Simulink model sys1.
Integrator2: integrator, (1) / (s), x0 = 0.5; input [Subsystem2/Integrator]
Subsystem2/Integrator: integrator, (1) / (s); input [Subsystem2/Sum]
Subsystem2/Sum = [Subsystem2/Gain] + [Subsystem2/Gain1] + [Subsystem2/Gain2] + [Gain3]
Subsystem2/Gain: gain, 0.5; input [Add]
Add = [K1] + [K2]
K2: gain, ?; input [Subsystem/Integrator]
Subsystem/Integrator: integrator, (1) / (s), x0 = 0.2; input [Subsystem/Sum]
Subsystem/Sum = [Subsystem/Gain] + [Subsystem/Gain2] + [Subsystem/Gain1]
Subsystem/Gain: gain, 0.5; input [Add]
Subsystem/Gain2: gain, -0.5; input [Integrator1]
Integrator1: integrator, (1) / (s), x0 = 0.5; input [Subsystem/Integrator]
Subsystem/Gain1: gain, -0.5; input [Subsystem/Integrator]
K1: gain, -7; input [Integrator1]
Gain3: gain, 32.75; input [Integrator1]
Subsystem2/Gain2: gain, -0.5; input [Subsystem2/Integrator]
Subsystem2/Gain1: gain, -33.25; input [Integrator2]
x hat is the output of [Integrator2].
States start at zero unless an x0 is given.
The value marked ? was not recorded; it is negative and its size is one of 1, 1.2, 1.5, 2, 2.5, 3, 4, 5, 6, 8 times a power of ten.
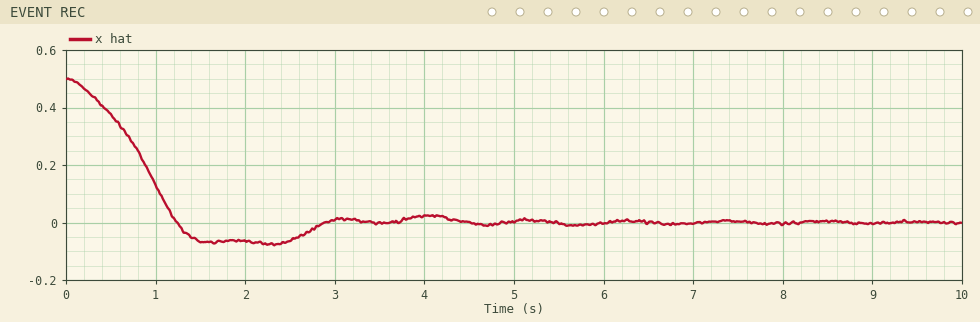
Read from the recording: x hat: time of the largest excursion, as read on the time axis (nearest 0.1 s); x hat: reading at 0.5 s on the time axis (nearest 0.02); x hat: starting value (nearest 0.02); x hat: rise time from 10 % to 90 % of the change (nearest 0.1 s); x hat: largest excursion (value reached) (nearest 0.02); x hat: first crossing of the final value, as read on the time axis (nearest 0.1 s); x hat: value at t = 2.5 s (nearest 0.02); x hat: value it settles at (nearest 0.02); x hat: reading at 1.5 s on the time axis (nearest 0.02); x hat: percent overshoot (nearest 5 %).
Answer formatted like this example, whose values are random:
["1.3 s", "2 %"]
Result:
["2.3 s", "0.38", "0.50", "0.9 s", "-0.08", "1.2 s", "-0.06", "0.00", "-0.06", "15 %"]
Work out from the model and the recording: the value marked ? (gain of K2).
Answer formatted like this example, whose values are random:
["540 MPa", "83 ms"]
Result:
["-3"]
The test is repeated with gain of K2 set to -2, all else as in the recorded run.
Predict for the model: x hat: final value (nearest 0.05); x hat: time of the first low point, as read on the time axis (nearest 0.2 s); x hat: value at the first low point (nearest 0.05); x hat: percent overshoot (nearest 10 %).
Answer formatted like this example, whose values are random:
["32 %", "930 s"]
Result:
["0.00", "1.6 s", "-0.15", "30 %"]
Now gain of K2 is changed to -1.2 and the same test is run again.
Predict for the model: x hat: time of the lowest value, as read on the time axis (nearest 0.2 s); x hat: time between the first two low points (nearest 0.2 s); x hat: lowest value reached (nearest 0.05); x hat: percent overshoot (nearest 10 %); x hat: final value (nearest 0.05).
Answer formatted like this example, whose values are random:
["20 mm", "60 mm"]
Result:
["1.6 s", "3.2 s", "-0.20", "40 %", "0.00"]
